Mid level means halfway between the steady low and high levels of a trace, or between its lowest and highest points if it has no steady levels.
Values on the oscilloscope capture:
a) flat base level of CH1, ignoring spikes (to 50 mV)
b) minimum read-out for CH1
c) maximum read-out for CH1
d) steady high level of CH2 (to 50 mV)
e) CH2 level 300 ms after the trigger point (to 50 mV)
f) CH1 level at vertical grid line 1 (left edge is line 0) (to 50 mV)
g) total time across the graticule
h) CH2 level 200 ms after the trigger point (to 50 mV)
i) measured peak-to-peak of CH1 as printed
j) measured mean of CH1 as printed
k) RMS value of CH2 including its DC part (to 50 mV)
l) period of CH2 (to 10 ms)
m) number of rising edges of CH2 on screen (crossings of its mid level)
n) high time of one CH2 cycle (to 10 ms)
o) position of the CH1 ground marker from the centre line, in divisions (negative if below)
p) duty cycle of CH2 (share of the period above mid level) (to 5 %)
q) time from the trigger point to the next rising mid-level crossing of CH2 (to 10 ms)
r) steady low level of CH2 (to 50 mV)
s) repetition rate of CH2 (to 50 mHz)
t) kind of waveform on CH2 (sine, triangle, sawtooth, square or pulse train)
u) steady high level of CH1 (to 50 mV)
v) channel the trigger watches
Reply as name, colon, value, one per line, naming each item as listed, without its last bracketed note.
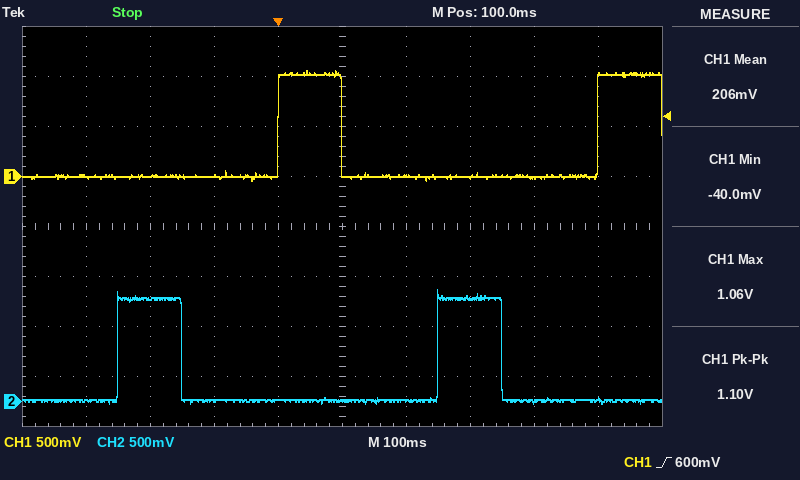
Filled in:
flat base level of CH1, ignoring spikes: 0 mV
minimum read-out for CH1: -40.0 mV
maximum read-out for CH1: 1.06 V
steady high level of CH2: 1.05 V
CH2 level 300 ms after the trigger point: 1.05 V
CH1 level at vertical grid line 1 (left edge is line 0): 0 mV
total time across the graticule: 1 s
CH2 level 200 ms after the trigger point: 0 mV
measured peak-to-peak of CH1 as printed: 1.10 V
measured mean of CH1 as printed: 206 mV
RMS value of CH2 including its DC part: 450 mV
period of CH2: 500 ms
number of rising edges of CH2 on screen: 2
high time of one CH2 cycle: 100 ms
position of the CH1 ground marker from the centre line, in divisions: +1.0 div
duty cycle of CH2 (share of the period above mid level): 20 %
time from the trigger point to the next rising mid-level crossing of CH2: 250 ms
steady low level of CH2: 0 mV
repetition rate of CH2: 2.00 Hz
kind of waveform on CH2: pulse train
steady high level of CH1: 1.00 V
channel the trigger watches: CH1
